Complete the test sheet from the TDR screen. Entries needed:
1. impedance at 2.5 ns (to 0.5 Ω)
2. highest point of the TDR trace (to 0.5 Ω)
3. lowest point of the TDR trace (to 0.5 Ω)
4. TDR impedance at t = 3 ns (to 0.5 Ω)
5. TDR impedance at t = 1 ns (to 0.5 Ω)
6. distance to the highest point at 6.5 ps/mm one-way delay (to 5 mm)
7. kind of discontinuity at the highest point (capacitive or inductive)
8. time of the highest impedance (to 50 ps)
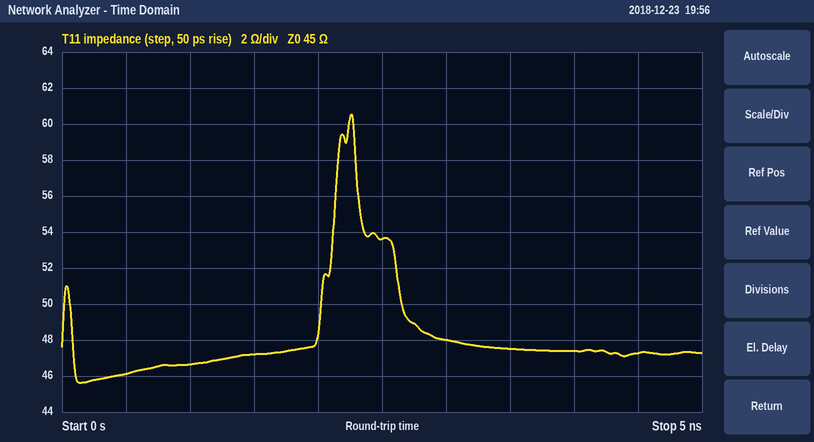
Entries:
53.5 Ω
60.5 Ω
45.5 Ω
48.0 Ω
46.5 Ω
175 mm
inductive
2.25 ns
